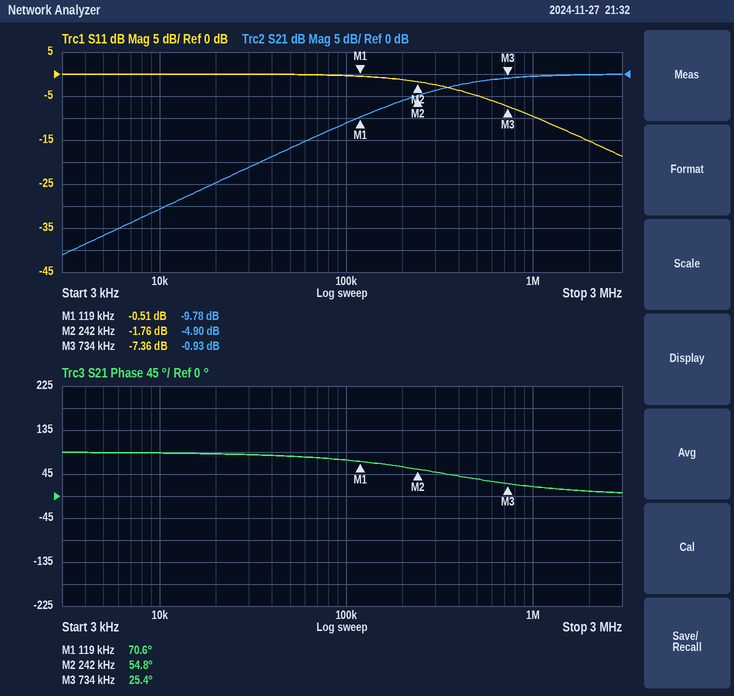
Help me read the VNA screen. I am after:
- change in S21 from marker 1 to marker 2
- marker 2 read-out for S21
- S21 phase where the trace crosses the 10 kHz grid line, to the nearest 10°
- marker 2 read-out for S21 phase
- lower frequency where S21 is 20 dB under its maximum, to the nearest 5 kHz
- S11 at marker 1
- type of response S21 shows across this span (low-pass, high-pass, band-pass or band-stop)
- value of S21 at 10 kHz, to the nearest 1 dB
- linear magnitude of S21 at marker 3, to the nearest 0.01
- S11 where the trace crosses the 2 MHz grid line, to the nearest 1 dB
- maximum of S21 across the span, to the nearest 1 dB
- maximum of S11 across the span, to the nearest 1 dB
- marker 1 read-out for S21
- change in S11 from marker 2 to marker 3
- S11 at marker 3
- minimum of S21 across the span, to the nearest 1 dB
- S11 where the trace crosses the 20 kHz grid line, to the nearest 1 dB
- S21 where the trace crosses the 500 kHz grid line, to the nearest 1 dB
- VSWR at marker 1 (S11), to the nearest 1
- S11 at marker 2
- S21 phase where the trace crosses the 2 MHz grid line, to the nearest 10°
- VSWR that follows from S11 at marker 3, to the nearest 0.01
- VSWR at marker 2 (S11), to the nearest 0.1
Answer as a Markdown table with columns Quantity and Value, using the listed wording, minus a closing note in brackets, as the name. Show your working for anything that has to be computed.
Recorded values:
| Quantity | Value |
|---|---|
| change in S21 from marker 1 to marker 2 | -4.9 − (-9.78) = 4.88 dB |
| marker 2 read-out for S21 | -4.90 dB |
| S21 phase where the trace crosses the 10 kHz grid line, to the nearest 10° | 90° |
| marker 2 read-out for S21 phase | 54.8° |
| lower frequency where S21 is 20 dB under its maximum, to the nearest 5 kHz | 35 kHz |
| S11 at marker 1 | -0.51 dB |
| type of response S21 shows across this span | high-pass |
| value of S21 at 10 kHz, to the nearest 1 dB | -31 dB |
| linear magnitude of S21 at marker 3, to the nearest 0.01 | 10^(-0.93/20) ≈ 0.90 |
| S11 where the trace crosses the 2 MHz grid line, to the nearest 1 dB | -15 dB |
| maximum of S21 across the span, to the nearest 1 dB | 0 dB |
| maximum of S11 across the span, to the nearest 1 dB | 0 dB |
| marker 1 read-out for S21 | -9.78 dB |
| change in S11 from marker 2 to marker 3 | -7.36 − (-1.76) = -5.60 dB |
| S11 at marker 3 | -7.36 dB |
| minimum of S21 across the span, to the nearest 1 dB | -41 dB |
| S11 where the trace crosses the 20 kHz grid line, to the nearest 1 dB | 0 dB |
| S21 where the trace crosses the 500 kHz grid line, to the nearest 1 dB | -2 dB |
| VSWR at marker 1 (S11), to the nearest 1 | (1 + 0.9430)/(1 − 0.9430) ≈ 34 |
| S11 at marker 2 | -1.76 dB |
| S21 phase where the trace crosses the 2 MHz grid line, to the nearest 10° | 10° |
| VSWR that follows from S11 at marker 3, to the nearest 0.01 | (1 + 0.4285)/(1 − 0.4285) ≈ 2.50 |
| VSWR at marker 2 (S11), to the nearest 0.1 | (1 + 0.8166)/(1 − 0.8166) ≈ 9.9 |
